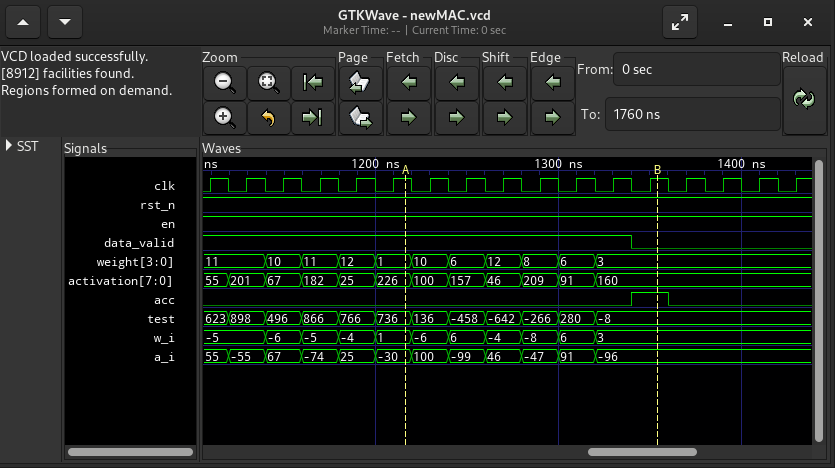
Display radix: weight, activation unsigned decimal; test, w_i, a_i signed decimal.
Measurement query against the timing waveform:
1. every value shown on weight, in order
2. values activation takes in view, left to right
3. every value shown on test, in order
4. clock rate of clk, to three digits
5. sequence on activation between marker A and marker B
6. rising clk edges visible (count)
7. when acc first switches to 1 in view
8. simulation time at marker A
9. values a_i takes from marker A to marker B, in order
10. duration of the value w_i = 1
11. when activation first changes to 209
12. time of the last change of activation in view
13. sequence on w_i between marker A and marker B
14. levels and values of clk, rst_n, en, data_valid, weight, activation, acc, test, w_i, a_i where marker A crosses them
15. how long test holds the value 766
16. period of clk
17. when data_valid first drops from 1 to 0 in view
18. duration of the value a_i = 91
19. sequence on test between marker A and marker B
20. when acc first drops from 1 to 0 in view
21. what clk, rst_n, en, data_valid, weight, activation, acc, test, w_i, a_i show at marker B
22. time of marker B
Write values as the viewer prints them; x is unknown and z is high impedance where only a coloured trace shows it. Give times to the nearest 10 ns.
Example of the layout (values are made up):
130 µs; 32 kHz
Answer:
11, 10, 11, 12, 1, 10, 6, 12, 8, 6, 3; 55, 201, 67, 182, 25, 226, 100, 157, 46, 209, 91, 160; 623, 898, 496, 866, 766, 736, 136, -458, -642, -266, 280, -8; 50.0 MHz; 226, 100, 157, 46, 209, 91, 160; 17; 1340 ns; 1220 ns; -30, 100, -99, 46, -47, 91, -96; 20 ns; 1280 ns; 1320 ns; 1, -6, 6, -4, -8, 6, 3; clk=1, rst_n=1, en=1, data_valid=1, weight=1, activation=226, acc=0, test=736, w_i=1, a_i=-30; 20 ns; 20 ns; 1340 ns; 20 ns; 736, 136, -458, -642, -266, 280, -8; 1360 ns; clk=1, rst_n=1, en=1, data_valid=0, weight=3, activation=160, acc=1, test=-8, w_i=3, a_i=-96; 1350 ns
